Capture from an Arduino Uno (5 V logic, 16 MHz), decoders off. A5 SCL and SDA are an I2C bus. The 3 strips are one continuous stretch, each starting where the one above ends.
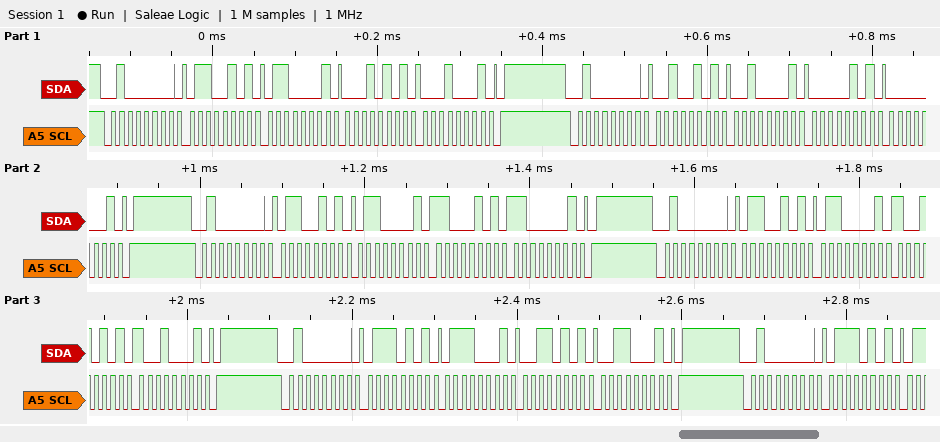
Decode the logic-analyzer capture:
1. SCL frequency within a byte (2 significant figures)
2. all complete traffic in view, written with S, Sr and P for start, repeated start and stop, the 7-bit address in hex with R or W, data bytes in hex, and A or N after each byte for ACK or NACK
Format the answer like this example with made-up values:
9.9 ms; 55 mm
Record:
100 kHz; S 20W A 65 A 61 A 15 A 11 A P S 20W A 25 A 21 A 05 A 01 A P S 20W A 65 A 61 A C5 A C1 A P S 20W A 65 A 61 A 95 A 91 A P S 20W A 75 A 71 A 35 A 31 A P S 20W A 75 A
